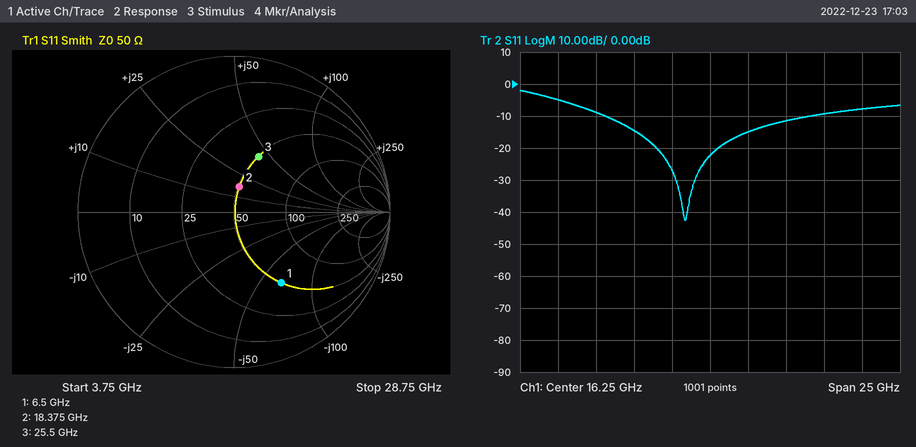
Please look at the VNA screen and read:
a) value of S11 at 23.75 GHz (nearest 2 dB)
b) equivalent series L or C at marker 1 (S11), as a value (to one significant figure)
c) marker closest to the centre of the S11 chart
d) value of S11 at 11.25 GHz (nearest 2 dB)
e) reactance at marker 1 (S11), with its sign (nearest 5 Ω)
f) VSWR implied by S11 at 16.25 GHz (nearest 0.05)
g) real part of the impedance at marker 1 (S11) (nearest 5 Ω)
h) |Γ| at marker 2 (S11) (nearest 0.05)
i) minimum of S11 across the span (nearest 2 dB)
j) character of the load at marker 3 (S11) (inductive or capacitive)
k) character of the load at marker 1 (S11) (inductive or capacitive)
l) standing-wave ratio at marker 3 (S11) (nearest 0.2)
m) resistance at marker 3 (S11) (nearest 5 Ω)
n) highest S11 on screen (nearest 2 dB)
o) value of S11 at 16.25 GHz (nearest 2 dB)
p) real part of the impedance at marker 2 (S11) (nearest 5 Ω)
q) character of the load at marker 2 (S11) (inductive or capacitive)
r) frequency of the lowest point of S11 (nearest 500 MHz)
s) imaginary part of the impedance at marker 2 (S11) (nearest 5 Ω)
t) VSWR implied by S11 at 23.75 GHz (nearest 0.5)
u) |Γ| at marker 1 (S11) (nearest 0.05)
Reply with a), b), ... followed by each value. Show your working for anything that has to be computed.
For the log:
a) -10 dB
b) C = 1/(2π × 6.5 GHz × 65 Ω) ≈ 377 fF, so 400 fF to one significant figure
c) marker 2
d) -14 dB
e) -65 Ω
f) |Γ| = 10^(-22/20) = 0.0794; VSWR = (1 + 0.0794)/(1 − 0.0794) ≈ 1.17, so 1.15 to the nearest 0.05
g) 50 Ω
h) 0.15
i) -42 dB
j) inductive
k) capacitive
l) 2.2
m) 50 Ω
n) -2 dB
o) -22 dB
p) 50 Ω
q) inductive
r) 14.5 GHz
s) +15 Ω
t) |Γ| = 10^(-10/20) = 0.3162; VSWR = (1 + 0.3162)/(1 − 0.3162) ≈ 1.92, so 2.0 to the nearest 0.5
u) 0.55
